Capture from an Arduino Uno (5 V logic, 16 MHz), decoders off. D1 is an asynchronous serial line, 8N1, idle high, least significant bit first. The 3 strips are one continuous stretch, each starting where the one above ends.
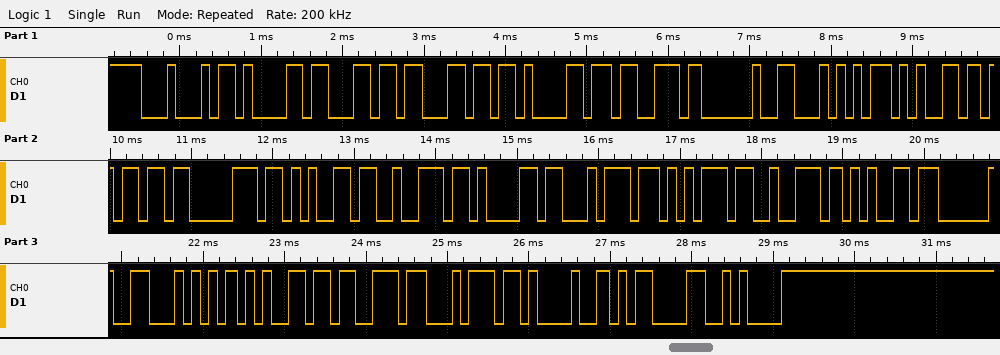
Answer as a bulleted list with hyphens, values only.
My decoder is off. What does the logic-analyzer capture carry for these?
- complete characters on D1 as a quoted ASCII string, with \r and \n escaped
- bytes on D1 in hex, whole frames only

- "Dallas Temperature Test!\r\n"
- 44 61 6C 6C 61 73 20 54 65 6D 70 65 72 61 74 75 72 65 20 54 65 73 74 21 0D 0A
